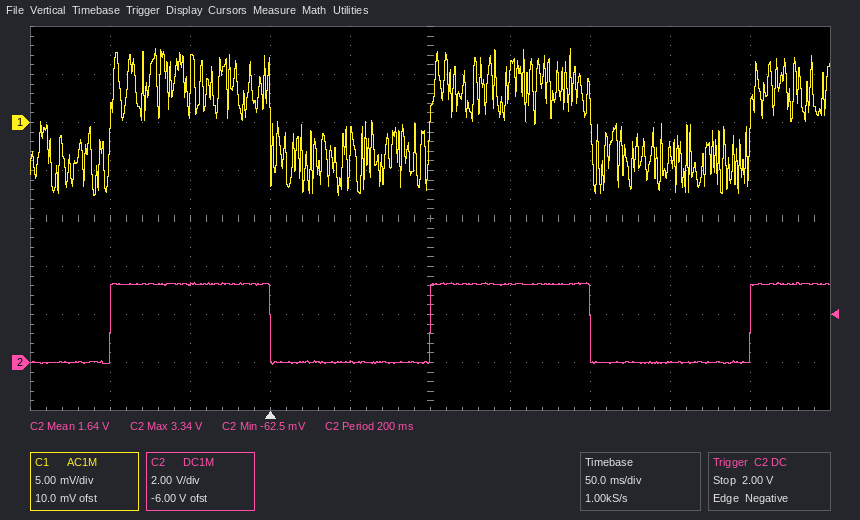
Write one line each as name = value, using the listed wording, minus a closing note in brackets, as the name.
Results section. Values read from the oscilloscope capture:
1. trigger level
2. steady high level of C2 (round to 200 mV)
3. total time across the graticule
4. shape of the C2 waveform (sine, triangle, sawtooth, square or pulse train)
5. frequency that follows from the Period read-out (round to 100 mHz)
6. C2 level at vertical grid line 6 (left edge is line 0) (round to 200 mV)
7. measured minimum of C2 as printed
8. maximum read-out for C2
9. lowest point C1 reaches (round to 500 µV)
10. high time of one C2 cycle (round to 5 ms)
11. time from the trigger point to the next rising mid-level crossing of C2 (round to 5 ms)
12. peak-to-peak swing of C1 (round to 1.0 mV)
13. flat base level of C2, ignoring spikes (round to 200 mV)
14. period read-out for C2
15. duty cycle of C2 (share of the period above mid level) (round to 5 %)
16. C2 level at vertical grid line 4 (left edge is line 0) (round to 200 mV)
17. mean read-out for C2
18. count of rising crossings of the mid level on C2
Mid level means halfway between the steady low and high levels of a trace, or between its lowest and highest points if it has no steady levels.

trigger level = 2.00 V
steady high level of C2 = 3.2 V
total time across the graticule = 500 ms
shape of the C2 waveform = square
frequency that follows from the Period read-out = 5.0 Hz
C2 level at vertical grid line 6 (left edge is line 0) = 3.2 V
measured minimum of C2 as printed = -62.5 mV
maximum read-out for C2 = 3.34 V
lowest point C1 reaches = -7.5 mV
high time of one C2 cycle = 100 ms
time from the trigger point to the next rising mid-level crossing of C2 = 100 ms
peak-to-peak swing of C1 = 15.0 mV
flat base level of C2, ignoring spikes = 0.0 V
period read-out for C2 = 200 ms
duty cycle of C2 (share of the period above mid level) = 50 %
C2 level at vertical grid line 4 (left edge is line 0) = 0.0 V
mean read-out for C2 = 1.64 V
count of rising crossings of the mid level on C2 = 3
